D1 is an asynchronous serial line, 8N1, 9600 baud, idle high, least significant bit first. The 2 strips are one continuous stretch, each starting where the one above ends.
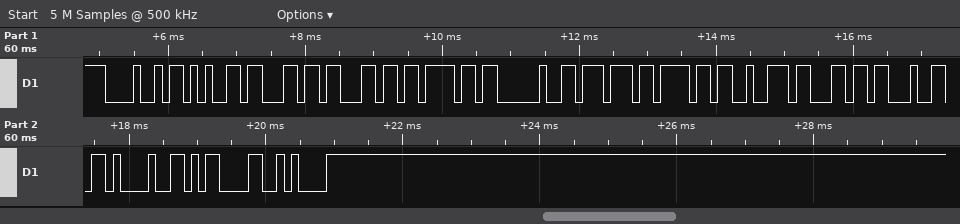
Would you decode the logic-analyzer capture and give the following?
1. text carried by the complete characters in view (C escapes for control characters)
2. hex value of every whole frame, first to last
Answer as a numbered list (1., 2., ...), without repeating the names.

1. "Hello world!\r\n"
2. 48 65 6C 6C 6F 20 77 6F 72 6C 64 21 0D 0A
